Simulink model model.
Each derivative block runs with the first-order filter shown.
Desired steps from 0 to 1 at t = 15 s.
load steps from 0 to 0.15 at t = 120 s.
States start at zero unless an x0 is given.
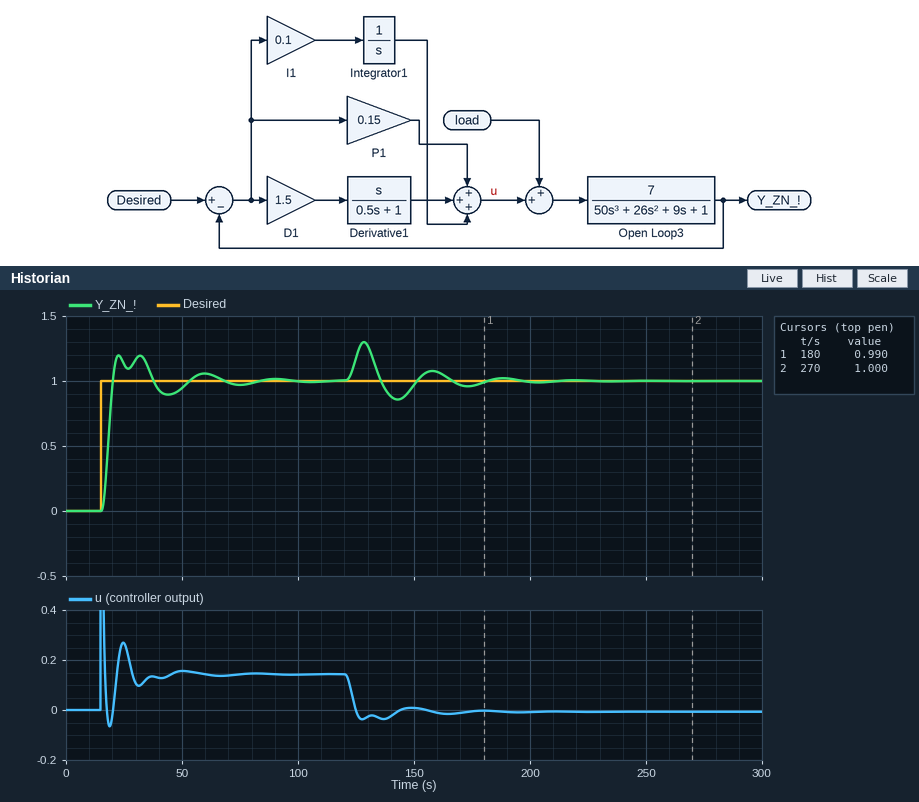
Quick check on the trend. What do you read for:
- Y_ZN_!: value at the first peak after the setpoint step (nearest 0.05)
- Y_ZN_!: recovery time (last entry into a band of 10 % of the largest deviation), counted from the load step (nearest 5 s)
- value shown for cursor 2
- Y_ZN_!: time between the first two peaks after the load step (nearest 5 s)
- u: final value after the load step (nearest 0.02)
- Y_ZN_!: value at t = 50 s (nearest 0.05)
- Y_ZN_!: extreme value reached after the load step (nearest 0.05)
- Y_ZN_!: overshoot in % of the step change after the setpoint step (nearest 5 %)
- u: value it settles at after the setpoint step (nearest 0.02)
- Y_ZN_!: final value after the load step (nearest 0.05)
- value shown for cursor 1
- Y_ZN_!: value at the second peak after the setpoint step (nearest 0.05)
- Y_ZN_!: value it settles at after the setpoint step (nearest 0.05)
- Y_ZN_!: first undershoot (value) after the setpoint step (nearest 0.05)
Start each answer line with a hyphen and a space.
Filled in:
- 1.20
- 55 s
- 1.000
- 30 s
- 0.00
- 0.95
- 1.30
- 20 %
- 0.14
- 1.00
- 0.990
- 1.20
- 1.00
- 1.10
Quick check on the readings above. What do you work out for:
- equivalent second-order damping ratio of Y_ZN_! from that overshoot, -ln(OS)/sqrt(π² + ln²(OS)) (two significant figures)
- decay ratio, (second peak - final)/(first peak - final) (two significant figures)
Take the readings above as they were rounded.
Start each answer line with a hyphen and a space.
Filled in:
- 0.46
- 1.0
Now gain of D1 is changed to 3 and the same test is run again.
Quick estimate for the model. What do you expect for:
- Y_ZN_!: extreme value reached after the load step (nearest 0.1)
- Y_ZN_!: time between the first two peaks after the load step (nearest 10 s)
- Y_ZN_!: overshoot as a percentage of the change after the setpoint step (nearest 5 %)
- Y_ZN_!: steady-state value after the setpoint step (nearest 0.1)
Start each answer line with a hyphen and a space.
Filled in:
- 1.2
- 40 s
- 25 %
- 1.0
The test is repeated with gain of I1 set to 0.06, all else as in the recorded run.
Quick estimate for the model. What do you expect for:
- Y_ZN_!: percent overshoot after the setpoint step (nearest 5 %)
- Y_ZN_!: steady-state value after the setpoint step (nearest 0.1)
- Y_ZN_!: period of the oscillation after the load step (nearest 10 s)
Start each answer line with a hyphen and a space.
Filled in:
- 15 %
- 1.0
- 40 s
